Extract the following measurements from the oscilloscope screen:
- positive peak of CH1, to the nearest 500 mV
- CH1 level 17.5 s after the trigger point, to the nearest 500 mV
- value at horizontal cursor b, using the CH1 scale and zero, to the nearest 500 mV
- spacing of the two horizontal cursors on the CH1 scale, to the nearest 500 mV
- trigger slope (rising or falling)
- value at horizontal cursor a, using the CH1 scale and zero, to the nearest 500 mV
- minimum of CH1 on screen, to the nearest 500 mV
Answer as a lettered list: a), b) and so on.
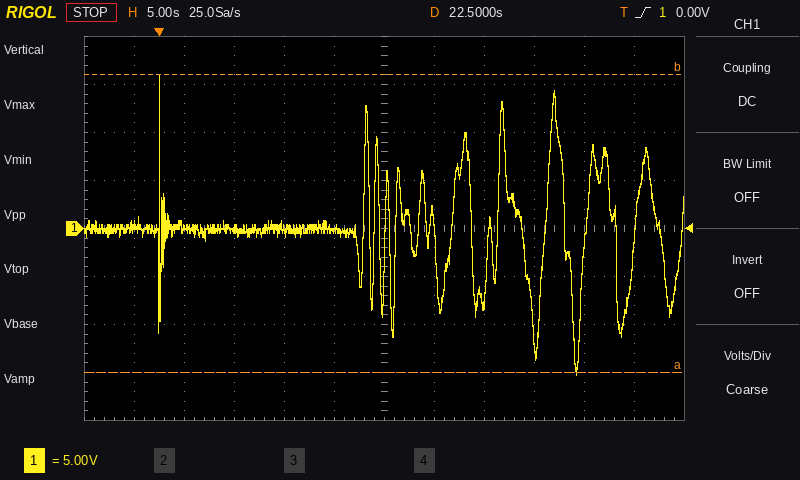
a) 16.0 V
b) 0.0 V
c) 16.0 V
d) 31.0 V
e) rising
f) -15.0 V
g) -15.0 V
